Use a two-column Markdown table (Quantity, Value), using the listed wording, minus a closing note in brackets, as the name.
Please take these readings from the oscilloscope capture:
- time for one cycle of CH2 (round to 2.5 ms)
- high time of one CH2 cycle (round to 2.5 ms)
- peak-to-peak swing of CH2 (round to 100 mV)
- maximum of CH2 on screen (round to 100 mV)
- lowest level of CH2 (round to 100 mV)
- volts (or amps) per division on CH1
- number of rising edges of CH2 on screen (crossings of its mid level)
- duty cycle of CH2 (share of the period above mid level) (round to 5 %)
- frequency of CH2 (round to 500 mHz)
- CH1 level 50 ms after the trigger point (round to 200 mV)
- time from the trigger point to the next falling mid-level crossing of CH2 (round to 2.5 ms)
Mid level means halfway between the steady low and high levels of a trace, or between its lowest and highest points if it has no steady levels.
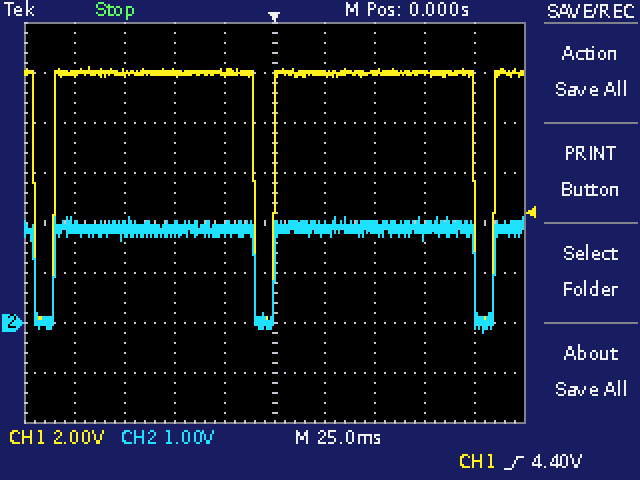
| Quantity | Value |
|---|---|
| time for one cycle of CH2 | 110.0 ms |
| high time of one CH2 cycle | 100.0 ms |
| peak-to-peak swing of CH2 | 2.3 V |
| maximum of CH2 on screen | 2.1 V |
| lowest level of CH2 | -200 mV |
| volts (or amps) per division on CH1 | 2 V |
| number of rising edges of CH2 on screen | 3 |
| duty cycle of CH2 (share of the period above mid level) | 90 % |
| frequency of CH2 | 9.0 Hz |
| CH1 level 50 ms after the trigger point | 10.0 V |
| time from the trigger point to the next falling mid-level crossing of CH2 | 100.0 ms |
